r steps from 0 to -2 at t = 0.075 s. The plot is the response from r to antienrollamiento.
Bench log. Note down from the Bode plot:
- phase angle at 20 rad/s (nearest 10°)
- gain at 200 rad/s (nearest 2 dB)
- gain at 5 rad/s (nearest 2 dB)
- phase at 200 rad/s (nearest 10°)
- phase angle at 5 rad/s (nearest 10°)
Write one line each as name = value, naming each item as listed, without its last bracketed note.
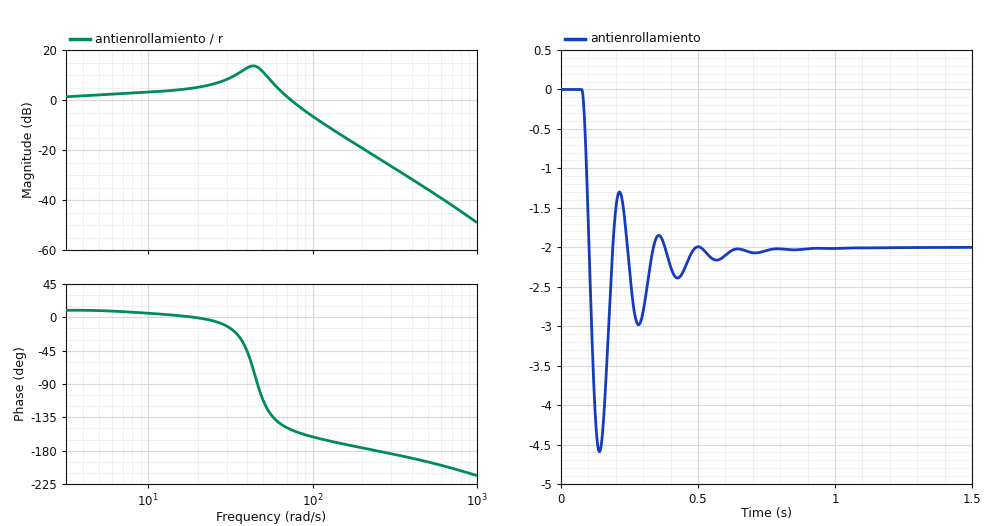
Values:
phase angle at 20 rad/s = 0°
gain at 200 rad/s = -20 dB
gain at 5 rad/s = 2 dB
phase at 200 rad/s = -180°
phase angle at 5 rad/s = 10°
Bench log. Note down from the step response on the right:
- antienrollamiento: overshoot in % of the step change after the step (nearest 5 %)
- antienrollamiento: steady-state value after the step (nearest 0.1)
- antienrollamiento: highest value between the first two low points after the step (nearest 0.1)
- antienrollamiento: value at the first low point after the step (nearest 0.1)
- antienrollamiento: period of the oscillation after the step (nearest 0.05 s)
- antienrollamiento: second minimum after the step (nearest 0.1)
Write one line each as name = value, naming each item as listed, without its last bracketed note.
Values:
antienrollamiento: overshoot in % of the step change after the step = 130 %
antienrollamiento: steady-state value after the step = -2.0
antienrollamiento: highest value between the first two low points after the step = -1.3
antienrollamiento: value at the first low point after the step = -4.6
antienrollamiento: period of the oscillation after the step = 0.15 s
antienrollamiento: second minimum after the step = -3.0
